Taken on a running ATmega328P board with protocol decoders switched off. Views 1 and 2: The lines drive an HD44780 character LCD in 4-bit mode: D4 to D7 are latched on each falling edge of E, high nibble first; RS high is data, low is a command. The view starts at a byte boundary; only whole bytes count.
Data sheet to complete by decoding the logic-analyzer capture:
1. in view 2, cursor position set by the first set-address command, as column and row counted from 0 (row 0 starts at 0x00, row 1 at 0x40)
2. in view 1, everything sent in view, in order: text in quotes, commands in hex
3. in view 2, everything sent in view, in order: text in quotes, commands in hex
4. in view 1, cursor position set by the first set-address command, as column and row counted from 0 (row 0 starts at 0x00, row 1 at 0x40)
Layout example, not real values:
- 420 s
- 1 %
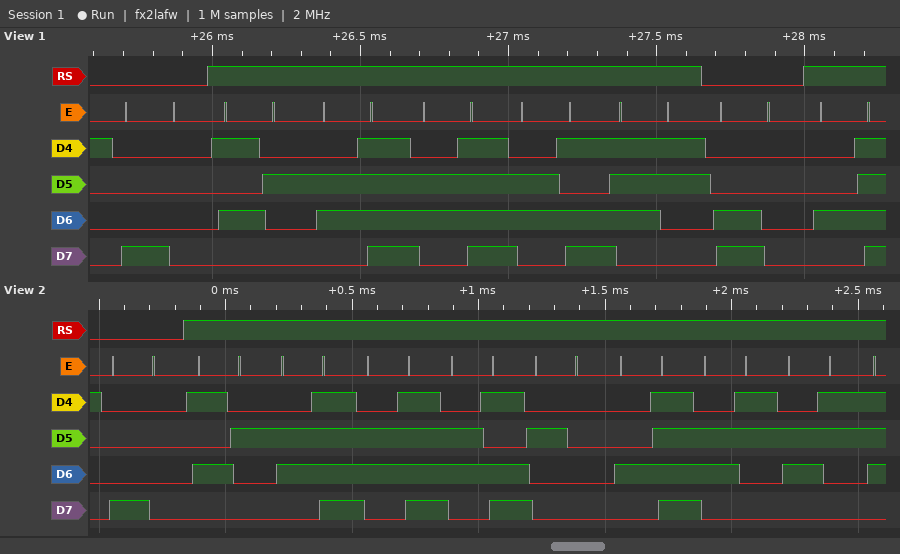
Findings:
- column 0, row 0
- 0x80 "Rooms" 0xC0 "O"
- 0x80 "Room Occ"
- column 0, row 0
